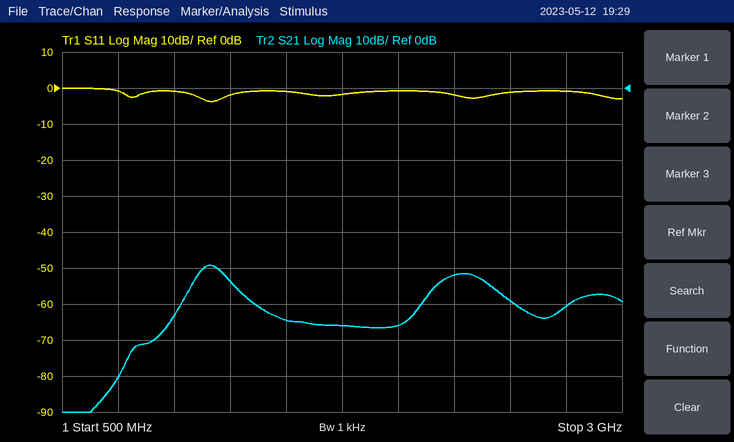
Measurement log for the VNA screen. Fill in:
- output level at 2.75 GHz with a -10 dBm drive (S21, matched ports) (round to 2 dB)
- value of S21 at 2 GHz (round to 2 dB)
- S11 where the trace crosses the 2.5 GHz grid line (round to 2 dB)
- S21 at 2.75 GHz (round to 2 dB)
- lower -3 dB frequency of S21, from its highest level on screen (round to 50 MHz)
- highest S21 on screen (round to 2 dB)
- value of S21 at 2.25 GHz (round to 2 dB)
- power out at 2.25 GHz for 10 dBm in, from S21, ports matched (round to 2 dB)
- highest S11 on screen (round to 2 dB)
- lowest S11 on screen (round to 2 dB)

-70 dBm
-66 dB
-2 dB
-60 dB
1.10 GHz
-50 dB
-52 dB
-42 dBm
0 dB
-4 dB
